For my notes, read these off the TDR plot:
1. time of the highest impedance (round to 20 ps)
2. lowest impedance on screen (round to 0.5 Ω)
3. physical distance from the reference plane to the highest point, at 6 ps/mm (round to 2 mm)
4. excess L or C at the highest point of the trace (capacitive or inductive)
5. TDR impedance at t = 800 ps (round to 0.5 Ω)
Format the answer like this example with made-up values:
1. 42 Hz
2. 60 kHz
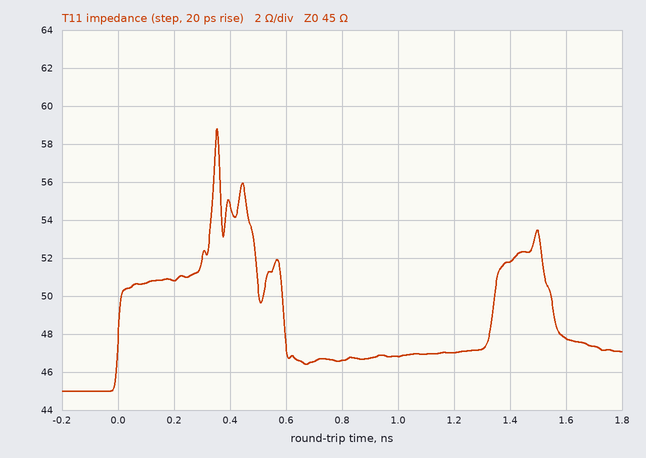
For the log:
1. 360 ps
2. 45.0 Ω
3. 30 mm
4. inductive
5. 46.5 Ω
